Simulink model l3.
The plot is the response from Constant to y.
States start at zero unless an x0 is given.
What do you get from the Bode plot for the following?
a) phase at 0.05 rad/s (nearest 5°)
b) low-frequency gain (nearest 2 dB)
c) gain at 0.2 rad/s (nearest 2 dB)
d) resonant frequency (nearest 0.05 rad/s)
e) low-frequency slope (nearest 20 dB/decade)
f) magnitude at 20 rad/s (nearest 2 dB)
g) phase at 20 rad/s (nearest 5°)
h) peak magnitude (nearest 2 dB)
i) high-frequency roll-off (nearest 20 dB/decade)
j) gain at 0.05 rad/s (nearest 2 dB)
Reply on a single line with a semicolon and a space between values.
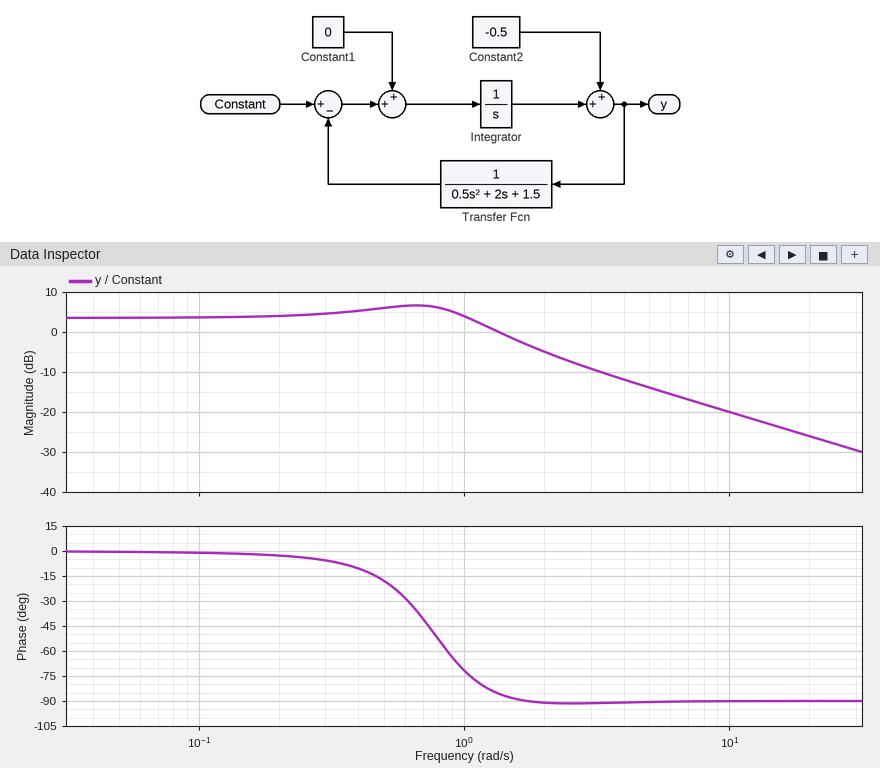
0°; 4 dB; 4 dB; 0.65 rad/s; 0 dB/decade; -26 dB; -90°; 6 dB; -20 dB/decade; 4 dB
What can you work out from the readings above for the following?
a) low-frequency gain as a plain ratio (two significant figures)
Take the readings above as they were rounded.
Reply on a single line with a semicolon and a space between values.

1.6
